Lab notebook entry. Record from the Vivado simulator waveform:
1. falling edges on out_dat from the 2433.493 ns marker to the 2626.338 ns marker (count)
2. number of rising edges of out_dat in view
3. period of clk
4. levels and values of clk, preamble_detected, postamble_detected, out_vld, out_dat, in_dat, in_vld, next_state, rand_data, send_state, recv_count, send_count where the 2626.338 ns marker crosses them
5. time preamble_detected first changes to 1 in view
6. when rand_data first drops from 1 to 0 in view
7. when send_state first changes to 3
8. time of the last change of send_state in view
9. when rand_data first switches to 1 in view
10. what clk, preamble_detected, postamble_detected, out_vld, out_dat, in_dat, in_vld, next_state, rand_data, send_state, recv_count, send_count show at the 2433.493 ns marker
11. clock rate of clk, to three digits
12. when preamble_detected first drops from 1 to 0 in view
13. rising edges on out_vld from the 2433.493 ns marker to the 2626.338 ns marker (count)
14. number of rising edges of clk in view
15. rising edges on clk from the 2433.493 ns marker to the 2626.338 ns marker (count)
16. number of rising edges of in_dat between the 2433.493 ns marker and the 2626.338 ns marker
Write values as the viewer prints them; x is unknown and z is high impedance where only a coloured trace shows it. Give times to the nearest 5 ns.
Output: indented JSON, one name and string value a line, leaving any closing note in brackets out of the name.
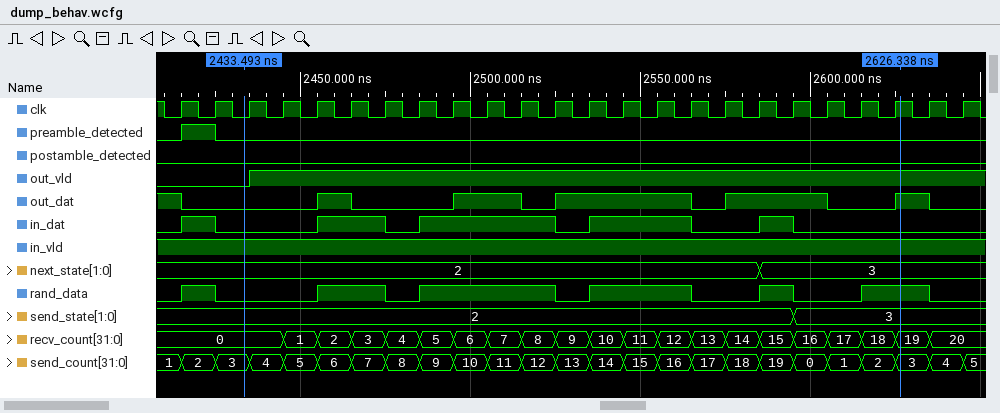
{
  "falling edges on out_dat from the 2433.493 ns marker to the 2626.338 ns marker": "4",
  "number of rising edges of out_dat in view": "5",
  "period of clk": "10 ns",
  "levels and values of clk, preamble_detected, postamble_detected, out_vld, out_dat, in_dat, in_vld, next_state, rand_data, send_state, recv_count, send_count where the 2626.338 ns marker crosses them": "clk=1, preamble_detected=0, postamble_detected=0, out_vld=1, out_dat=1, in_dat=0, in_vld=1, next_state=3, rand_data=1, send_state=3, recv_count=19, send_count=3",
  "time preamble_detected first changes to 1 in view": "2415 ns",
  "when rand_data first drops from 1 to 0 in view": "2425 ns",
  "when send_state first changes to 3": "2595 ns",
  "time of the last change of send_state in view": "2595 ns",
  "when rand_data first switches to 1 in view": "2415 ns",
  "what clk, preamble_detected, postamble_detected, out_vld, out_dat, in_dat, in_vld, next_state, rand_data, send_state, recv_count, send_count show at the 2433.493 ns marker": "clk=0, preamble_detected=0, postamble_detected=0, out_vld=0, out_dat=0, in_dat=0, in_vld=1, next_state=2, rand_data=0, send_state=2, recv_count=0, send_count=3",
  "clock rate of clk, to three digits": "100 MHz",
  "when preamble_detected first drops from 1 to 0 in view": "2425 ns",
  "rising edges on out_vld from the 2433.493 ns marker to the 2626.338 ns marker": "1",
  "number of rising edges of clk in view": "24",
  "rising edges on clk from the 2433.493 ns marker to the 2626.338 ns marker": "20",
  "number of rising edges of in_dat between the 2433.493 ns marker and the 2626.338 ns marker": "4"
}
